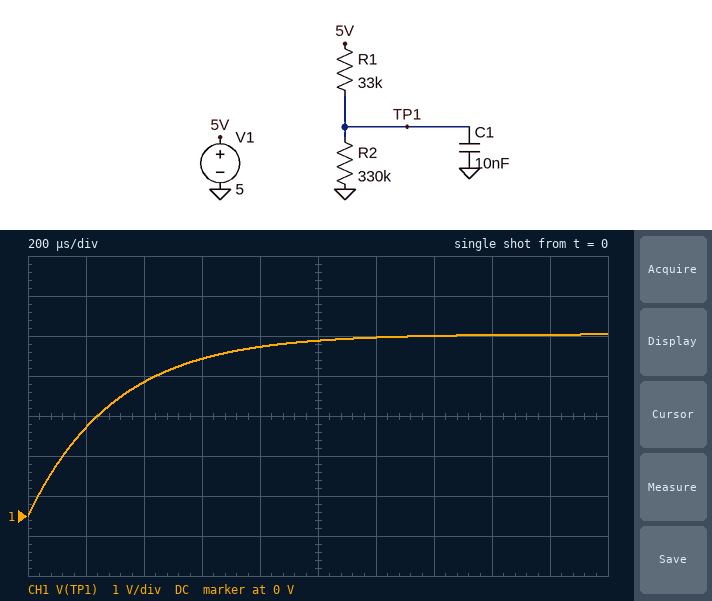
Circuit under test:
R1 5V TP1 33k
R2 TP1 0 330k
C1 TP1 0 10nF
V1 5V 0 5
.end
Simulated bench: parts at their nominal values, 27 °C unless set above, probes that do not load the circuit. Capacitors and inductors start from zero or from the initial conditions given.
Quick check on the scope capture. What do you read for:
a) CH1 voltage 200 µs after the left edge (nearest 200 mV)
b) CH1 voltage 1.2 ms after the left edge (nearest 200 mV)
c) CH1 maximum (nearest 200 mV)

2.2 V
4.4 V
4.6 V
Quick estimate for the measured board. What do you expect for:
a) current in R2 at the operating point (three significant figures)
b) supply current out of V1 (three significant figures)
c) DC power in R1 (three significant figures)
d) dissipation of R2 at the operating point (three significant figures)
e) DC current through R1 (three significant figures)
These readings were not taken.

13.8 µA
13.8 µA
6.26 µW
62.6 µW
13.8 µA
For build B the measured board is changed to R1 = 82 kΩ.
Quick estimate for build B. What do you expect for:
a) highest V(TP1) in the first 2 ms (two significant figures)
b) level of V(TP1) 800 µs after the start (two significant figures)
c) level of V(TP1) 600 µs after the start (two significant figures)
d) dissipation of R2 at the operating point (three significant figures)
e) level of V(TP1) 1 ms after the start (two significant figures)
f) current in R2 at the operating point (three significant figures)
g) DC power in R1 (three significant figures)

3.8 V
2.8 V
2.4 V
48.6 µW
3.1 V
12.1 µA
12.1 µW
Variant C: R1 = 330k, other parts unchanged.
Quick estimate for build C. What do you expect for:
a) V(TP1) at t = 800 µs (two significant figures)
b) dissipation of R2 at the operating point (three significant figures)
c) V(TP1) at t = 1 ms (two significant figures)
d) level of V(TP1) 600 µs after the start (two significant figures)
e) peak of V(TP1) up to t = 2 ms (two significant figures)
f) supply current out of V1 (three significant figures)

960 mV
18.9 µW
1.1 V
760 mV
1.8 V
7.58 µA
